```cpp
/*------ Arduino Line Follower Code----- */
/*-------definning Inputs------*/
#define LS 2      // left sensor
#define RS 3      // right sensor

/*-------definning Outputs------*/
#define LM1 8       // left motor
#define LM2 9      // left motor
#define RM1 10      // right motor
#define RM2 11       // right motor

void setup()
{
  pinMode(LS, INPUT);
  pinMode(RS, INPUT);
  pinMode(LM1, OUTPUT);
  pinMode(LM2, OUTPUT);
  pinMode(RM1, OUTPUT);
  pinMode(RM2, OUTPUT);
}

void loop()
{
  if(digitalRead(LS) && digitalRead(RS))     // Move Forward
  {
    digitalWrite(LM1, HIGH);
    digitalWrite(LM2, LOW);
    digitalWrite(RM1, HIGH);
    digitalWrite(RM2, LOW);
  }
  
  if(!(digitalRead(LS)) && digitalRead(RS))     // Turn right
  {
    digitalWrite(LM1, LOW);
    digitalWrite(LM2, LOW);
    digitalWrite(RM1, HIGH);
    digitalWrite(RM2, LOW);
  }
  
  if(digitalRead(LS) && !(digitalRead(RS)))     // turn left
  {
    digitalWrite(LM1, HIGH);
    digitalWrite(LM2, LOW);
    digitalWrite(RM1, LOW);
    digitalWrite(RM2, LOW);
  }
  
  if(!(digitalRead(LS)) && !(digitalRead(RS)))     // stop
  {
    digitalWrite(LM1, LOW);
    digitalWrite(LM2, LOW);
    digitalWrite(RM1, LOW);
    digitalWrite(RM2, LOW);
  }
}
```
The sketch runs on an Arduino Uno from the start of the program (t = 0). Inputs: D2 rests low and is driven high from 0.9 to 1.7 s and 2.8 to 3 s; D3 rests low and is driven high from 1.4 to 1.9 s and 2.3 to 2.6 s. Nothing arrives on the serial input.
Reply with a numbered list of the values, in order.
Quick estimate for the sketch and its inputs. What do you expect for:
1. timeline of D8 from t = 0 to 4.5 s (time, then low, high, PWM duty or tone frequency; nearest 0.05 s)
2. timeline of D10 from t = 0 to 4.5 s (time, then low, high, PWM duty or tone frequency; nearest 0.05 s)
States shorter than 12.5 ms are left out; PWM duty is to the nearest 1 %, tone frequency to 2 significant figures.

1. 0 s low; 0.9 s high; 1.7 s low; 2.8 s high; 3 s low
2. 0 s low; 1.4 s high; 1.9 s low; 2.3 s high; 2.6 s low
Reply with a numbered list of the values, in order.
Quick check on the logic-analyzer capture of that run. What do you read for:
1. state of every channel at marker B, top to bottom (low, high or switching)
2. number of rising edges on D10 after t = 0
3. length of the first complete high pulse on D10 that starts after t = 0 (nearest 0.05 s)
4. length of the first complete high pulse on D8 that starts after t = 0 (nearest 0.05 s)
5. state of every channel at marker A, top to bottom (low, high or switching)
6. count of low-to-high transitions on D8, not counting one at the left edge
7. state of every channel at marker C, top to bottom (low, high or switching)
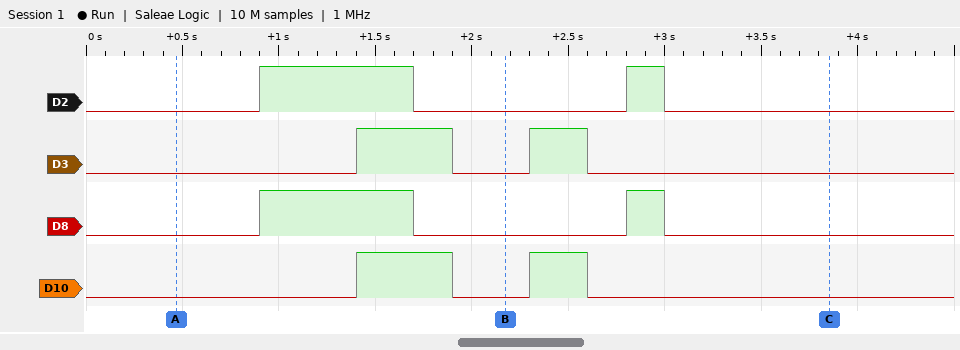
1. D2 low, D3 low, D8 low, D10 low
2. 2
3. 0.50 s
4. 0.80 s
5. D2 low, D3 low, D8 low, D10 low
6. 2
7. D2 low, D3 low, D8 low, D10 low
